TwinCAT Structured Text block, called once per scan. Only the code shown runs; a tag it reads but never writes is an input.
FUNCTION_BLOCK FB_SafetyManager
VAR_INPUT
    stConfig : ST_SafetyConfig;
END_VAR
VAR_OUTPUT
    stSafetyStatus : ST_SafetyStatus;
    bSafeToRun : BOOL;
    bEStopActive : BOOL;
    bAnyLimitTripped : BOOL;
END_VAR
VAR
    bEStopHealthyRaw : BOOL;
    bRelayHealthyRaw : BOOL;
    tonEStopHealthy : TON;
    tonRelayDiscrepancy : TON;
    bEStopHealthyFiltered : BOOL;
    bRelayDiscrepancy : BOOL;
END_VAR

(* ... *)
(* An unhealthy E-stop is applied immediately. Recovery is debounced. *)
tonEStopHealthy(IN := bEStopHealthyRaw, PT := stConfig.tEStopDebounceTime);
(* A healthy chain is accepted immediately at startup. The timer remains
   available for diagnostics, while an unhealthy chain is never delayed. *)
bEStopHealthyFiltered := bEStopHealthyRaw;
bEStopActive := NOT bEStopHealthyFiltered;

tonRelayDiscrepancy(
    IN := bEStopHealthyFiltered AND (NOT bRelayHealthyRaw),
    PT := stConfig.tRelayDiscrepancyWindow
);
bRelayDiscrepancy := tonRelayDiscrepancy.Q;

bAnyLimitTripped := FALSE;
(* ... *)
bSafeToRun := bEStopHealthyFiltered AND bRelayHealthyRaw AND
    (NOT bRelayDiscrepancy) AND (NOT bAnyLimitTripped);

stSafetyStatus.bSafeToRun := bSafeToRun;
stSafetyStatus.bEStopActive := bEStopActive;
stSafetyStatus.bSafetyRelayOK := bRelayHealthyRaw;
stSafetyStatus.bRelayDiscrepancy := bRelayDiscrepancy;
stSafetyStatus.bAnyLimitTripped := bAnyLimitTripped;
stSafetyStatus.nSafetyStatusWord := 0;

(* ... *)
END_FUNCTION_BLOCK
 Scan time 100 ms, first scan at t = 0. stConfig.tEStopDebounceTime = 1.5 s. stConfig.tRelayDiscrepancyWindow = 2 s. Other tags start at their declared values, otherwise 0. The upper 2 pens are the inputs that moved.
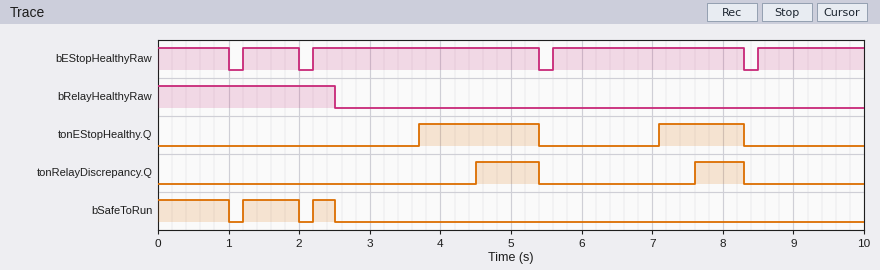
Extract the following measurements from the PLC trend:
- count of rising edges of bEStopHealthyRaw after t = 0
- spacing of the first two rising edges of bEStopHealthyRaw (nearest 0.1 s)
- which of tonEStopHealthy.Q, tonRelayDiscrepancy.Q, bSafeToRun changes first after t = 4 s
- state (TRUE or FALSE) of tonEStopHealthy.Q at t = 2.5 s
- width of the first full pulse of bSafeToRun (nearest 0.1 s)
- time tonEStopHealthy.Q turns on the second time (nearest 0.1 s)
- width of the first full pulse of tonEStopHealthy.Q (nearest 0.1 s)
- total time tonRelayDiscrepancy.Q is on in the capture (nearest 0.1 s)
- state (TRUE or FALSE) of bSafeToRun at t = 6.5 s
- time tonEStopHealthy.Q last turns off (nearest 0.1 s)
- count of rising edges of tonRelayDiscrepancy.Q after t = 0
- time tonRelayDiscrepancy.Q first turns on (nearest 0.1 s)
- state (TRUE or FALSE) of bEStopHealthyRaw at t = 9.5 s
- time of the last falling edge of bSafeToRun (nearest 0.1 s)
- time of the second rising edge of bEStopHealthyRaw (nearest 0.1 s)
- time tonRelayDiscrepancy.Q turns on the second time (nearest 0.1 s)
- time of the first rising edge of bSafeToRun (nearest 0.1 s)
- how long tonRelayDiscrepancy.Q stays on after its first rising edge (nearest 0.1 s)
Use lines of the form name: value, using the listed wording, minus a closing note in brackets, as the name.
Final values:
count of rising edges of bEStopHealthyRaw after t = 0: 4
spacing of the first two rising edges of bEStopHealthyRaw: 1.0 s
which of tonEStopHealthy.Q, tonRelayDiscrepancy.Q, bSafeToRun changes first after t = 4 s: tonRelayDiscrepancy.Q
state (TRUE or FALSE) of tonEStopHealthy.Q at t = 2.5 s: FALSE
width of the first full pulse of bSafeToRun: 0.8 s
time tonEStopHealthy.Q turns on the second time: 7.1 s
width of the first full pulse of tonEStopHealthy.Q: 1.7 s
total time tonRelayDiscrepancy.Q is on in the capture: 1.6 s
state (TRUE or FALSE) of bSafeToRun at t = 6.5 s: FALSE
time tonEStopHealthy.Q last turns off: 8.3 s
count of rising edges of tonRelayDiscrepancy.Q after t = 0: 2
time tonRelayDiscrepancy.Q first turns on: 4.5 s
state (TRUE or FALSE) of bEStopHealthyRaw at t = 9.5 s: TRUE
time of the last falling edge of bSafeToRun: 2.5 s
time of the second rising edge of bEStopHealthyRaw: 2.2 s
time tonRelayDiscrepancy.Q turns on the second time: 7.6 s
time of the first rising edge of bSafeToRun: 1.2 s
how long tonRelayDiscrepancy.Q stays on after its first rising edge: 0.9 s
